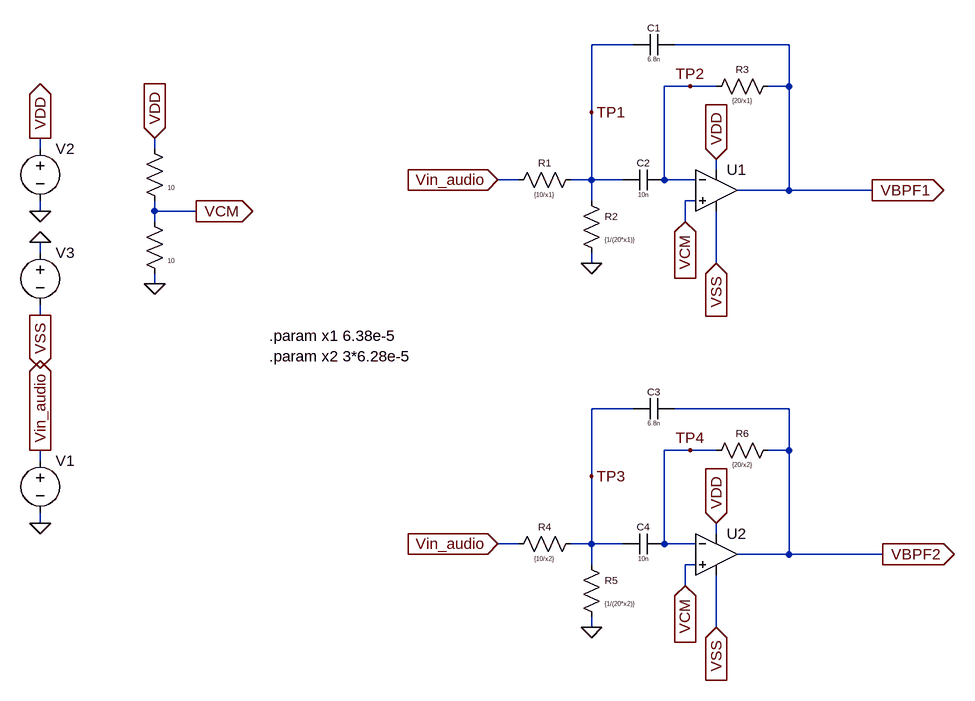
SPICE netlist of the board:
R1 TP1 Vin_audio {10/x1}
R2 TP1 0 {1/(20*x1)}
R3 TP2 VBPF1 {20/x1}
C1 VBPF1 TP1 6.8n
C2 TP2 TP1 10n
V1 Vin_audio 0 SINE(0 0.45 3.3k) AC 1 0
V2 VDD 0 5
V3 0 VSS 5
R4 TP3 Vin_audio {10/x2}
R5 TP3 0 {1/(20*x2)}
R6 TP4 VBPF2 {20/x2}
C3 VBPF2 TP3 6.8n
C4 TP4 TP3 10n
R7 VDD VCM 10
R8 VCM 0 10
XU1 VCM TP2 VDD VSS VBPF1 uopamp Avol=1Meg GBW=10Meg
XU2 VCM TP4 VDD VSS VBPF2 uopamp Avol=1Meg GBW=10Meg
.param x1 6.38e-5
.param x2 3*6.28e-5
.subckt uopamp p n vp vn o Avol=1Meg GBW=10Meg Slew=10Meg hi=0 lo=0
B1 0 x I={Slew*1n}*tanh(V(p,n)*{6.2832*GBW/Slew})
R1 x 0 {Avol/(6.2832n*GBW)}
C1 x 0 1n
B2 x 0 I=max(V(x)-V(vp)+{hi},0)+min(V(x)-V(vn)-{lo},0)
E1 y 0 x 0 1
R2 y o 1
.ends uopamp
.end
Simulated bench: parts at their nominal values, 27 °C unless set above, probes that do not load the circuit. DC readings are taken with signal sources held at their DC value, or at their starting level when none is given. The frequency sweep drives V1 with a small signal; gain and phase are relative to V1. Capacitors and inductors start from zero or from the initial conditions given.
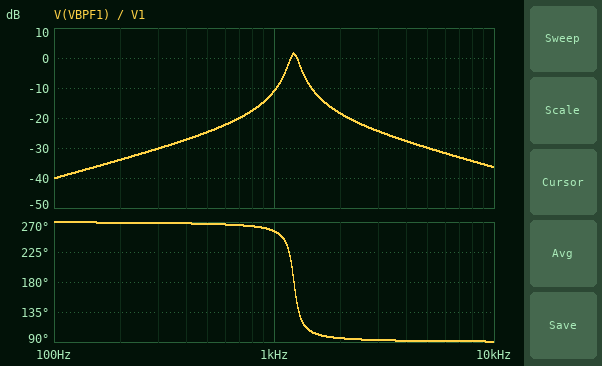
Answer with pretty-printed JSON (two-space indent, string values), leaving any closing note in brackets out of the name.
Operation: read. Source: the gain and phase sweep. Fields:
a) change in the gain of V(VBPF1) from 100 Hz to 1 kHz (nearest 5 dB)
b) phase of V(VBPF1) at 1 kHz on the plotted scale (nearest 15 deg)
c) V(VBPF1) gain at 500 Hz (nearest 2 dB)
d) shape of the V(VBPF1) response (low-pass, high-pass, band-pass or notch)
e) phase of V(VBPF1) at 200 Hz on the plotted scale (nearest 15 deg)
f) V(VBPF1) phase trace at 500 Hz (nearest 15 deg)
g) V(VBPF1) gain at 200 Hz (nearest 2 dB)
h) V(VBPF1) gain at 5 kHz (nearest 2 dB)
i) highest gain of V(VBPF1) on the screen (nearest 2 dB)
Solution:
{
  "change in the gain of V(VBPF1) from 100 Hz to 1 kHz": "30 dB",
  "phase of V(VBPF1) at 1 kHz on the plotted scale": "255 deg",
  "V(VBPF1) gain at 500 Hz": "-24 dB",
  "shape of the V(VBPF1) response": "band-pass",
  "phase of V(VBPF1) at 200 Hz on the plotted scale": "270 deg",
  "V(VBPF1) phase trace at 500 Hz": "270 deg",
  "V(VBPF1) gain at 200 Hz": "-34 dB",
  "V(VBPF1) gain at 5 kHz": "-30 dB",
  "highest gain of V(VBPF1) on the screen": "2 dB"
}
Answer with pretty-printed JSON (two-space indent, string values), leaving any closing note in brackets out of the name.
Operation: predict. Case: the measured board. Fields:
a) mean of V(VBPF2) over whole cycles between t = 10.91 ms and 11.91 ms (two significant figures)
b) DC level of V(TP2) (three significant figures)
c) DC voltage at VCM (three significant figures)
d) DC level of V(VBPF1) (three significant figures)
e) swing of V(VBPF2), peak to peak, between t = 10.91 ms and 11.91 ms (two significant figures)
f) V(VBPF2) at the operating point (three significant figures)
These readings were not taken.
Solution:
{
  "mean of V(VBPF2) over whole cycles between t = 10.91 ms and 11.91 ms": "2.5 V",
  "DC level of V(TP2)": "2.50 V",
  "DC voltage at VCM": "2.50 V",
  "DC level of V(VBPF1)": "2.50 V",
  "swing of V(VBPF2), peak to peak, between t = 10.91 ms and 11.91 ms": "500 mV",
  "V(VBPF2) at the operating point": "2.50 V"
}
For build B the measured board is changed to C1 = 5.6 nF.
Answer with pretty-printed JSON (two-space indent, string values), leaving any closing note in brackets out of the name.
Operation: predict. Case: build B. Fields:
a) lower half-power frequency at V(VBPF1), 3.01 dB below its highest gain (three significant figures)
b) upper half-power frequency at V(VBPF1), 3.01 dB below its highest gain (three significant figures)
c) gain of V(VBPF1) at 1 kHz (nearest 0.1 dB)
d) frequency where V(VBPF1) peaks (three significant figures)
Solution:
{
  "lower half-power frequency at V(VBPF1), 3.01 dB below its highest gain": "1.29 kHz",
  "upper half-power frequency at V(VBPF1), 3.01 dB below its highest gain": "1.43 kHz",
  "gain of V(VBPF1) at 1 kHz": "-13.5 dB",
  "frequency where V(VBPF1) peaks": "1.36 kHz"
}
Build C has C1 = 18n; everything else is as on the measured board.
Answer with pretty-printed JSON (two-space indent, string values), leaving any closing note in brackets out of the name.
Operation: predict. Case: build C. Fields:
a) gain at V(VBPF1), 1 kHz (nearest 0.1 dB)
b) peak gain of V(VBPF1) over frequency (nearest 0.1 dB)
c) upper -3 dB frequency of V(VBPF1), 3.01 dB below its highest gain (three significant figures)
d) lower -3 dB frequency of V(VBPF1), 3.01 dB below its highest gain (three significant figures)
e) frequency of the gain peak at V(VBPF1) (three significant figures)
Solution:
{
  "gain at V(VBPF1), 1 kHz": "-17.7 dB",
  "peak gain of V(VBPF1) over frequency": "-2.9 dB",
  "upper -3 dB frequency of V(VBPF1), 3.01 dB below its highest gain": "799 Hz",
  "lower -3 dB frequency of V(VBPF1), 3.01 dB below its highest gain": "720 Hz",
  "frequency of the gain peak at V(VBPF1)": "758 Hz"
}
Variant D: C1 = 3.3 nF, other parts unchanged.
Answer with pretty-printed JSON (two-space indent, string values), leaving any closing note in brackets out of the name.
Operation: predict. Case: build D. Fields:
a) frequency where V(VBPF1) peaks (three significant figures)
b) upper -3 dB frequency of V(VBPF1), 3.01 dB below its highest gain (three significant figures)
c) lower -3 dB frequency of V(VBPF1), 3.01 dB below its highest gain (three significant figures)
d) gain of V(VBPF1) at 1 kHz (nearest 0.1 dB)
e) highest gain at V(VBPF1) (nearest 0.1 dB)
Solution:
{
  "frequency where V(VBPF1) peaks": "1.77 kHz",
  "upper -3 dB frequency of V(VBPF1), 3.01 dB below its highest gain": "1.87 kHz",
  "lower -3 dB frequency of V(VBPF1), 3.01 dB below its highest gain": "1.67 kHz",
  "gain of V(VBPF1) at 1 kHz": "-16.9 dB",
  "highest gain at V(VBPF1)": "3.5 dB"
}
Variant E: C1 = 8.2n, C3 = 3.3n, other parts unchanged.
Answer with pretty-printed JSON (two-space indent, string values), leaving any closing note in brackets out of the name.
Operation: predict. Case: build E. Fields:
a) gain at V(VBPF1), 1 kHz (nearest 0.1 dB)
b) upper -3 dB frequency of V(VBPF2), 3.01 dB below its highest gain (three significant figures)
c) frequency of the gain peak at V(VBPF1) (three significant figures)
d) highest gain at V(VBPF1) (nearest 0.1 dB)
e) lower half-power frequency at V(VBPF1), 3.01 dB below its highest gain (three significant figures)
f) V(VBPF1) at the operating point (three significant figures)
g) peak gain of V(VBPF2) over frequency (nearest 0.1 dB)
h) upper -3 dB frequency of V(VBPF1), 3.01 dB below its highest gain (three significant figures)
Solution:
{
  "gain at V(VBPF1), 1 kHz": "-7.2 dB",
  "upper -3 dB frequency of V(VBPF2), 3.01 dB below its highest gain": "5.49 kHz",
  "frequency of the gain peak at V(VBPF1)": "1.12 kHz",
  "highest gain at V(VBPF1)": "0.8 dB",
  "lower half-power frequency at V(VBPF1), 3.01 dB below its highest gain": "1.07 kHz",
  "V(VBPF1) at the operating point": "2.50 V",
  "peak gain of V(VBPF2) over frequency": "3.5 dB",
  "upper -3 dB frequency of V(VBPF1), 3.01 dB below its highest gain": "1.18 kHz"
}
